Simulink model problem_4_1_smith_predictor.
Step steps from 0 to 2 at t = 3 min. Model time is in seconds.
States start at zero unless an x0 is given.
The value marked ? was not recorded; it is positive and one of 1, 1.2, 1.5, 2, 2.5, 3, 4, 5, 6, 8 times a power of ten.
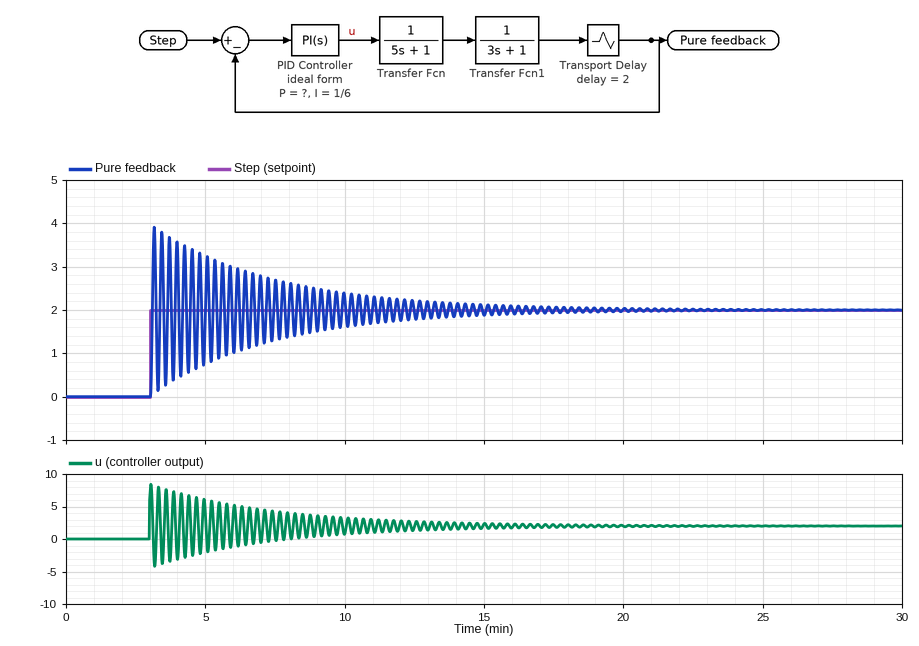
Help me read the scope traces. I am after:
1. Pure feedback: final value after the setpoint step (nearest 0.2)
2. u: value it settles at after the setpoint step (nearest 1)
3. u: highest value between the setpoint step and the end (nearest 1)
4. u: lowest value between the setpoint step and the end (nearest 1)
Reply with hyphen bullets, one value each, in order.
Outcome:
- 2.0
- 2
- 8
- -4
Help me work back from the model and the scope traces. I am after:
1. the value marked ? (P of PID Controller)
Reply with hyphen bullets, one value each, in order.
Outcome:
- 3
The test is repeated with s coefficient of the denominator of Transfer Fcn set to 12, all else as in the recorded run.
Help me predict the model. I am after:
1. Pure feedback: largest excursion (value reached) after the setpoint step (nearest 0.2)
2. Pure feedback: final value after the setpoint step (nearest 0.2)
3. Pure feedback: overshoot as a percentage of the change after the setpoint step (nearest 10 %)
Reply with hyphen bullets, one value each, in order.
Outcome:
- 3.6
- 2.0
- 80 %
